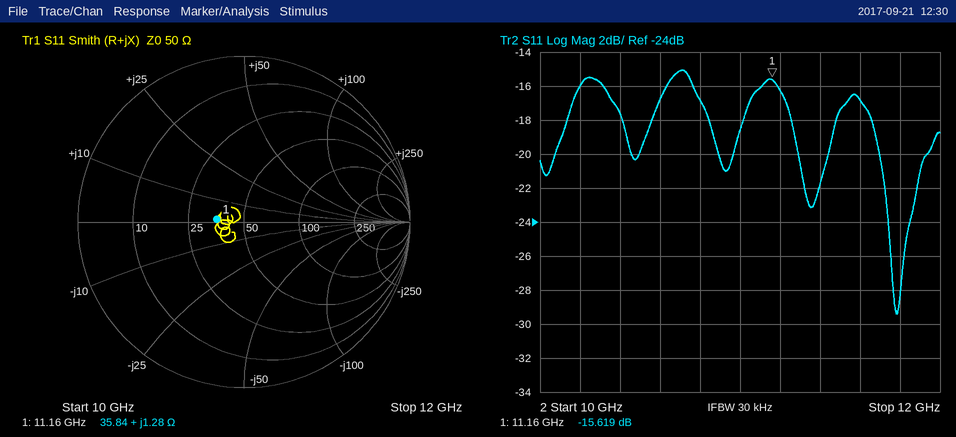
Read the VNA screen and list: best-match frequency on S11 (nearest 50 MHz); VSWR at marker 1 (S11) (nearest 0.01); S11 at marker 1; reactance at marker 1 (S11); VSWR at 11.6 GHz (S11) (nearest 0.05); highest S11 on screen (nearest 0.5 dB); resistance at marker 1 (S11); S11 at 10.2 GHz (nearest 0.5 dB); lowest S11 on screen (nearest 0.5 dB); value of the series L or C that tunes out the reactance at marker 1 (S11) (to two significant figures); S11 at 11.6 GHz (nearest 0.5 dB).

11.80 GHz
1.40
-15.619 dB
+1.28 Ω
1.35
-15.0 dB
35.84 Ω
-16.0 dB
-29.5 dB
11 pF
-17.0 dB
